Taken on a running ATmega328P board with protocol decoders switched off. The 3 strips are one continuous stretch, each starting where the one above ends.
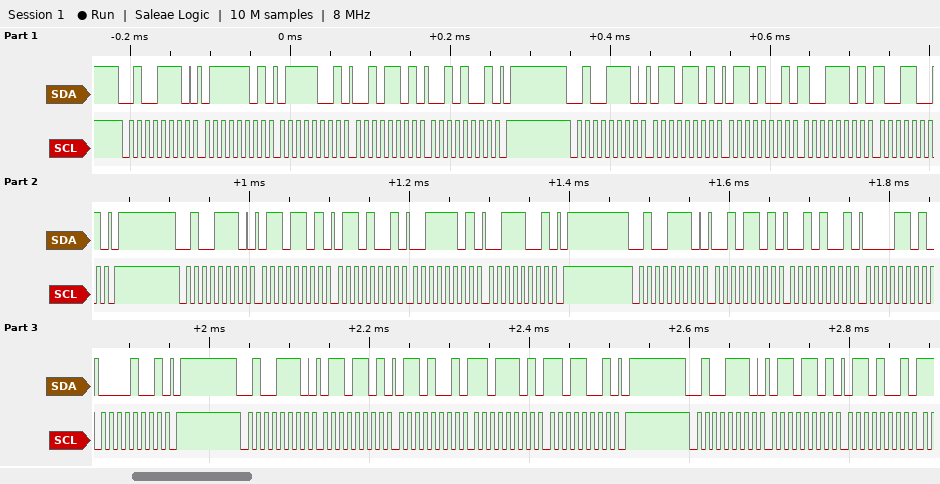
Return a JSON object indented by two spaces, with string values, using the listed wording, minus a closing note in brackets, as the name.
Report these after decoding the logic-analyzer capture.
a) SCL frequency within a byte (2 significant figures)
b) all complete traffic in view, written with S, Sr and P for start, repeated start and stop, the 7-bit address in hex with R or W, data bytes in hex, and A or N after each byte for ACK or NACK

{
  "SCL frequency within a byte": "100 kHz",
  "all complete traffic in view, written with S, Sr and P for start, repeated start and stop, the 7-bit address in hex with R or W, data bytes in hex, and A or N after each byte for ACK or NACK": "S 27W A 7D A 79 A 2D A 29 A P S 27W A 6D A 69 A 9D A 99 A P S 27W A 6D A 69 A 3D A 39 A P S 27W A 2D A 29 A 0D A 09 A P S 27W A 6D A 69 A DD A D9 A P S 27W A 6D A 69 A"
}
